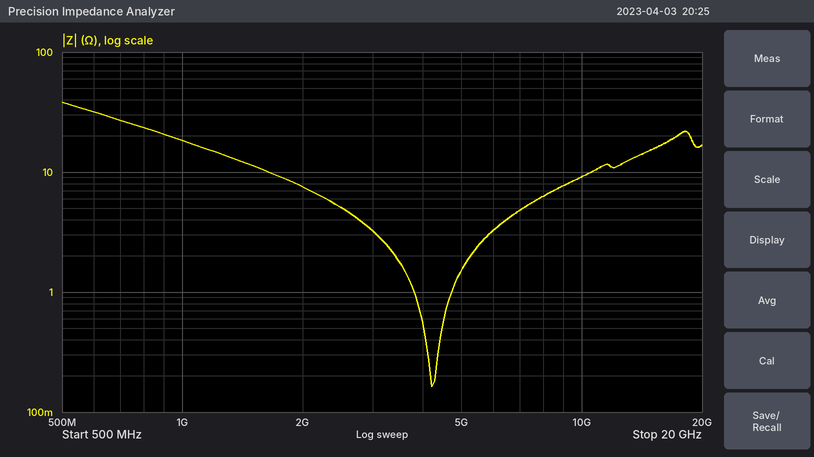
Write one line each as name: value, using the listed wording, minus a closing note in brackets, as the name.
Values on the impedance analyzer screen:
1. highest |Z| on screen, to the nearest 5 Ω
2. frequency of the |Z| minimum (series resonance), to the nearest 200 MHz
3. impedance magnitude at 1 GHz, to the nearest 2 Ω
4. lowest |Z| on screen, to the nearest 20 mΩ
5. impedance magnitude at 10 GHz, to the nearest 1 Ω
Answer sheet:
highest |Z| on screen, to the nearest 5 Ω: 40 Ω
frequency of the |Z| minimum (series resonance), to the nearest 200 MHz: 4.2 GHz
impedance magnitude at 1 GHz, to the nearest 2 Ω: 18 Ω
lowest |Z| on screen, to the nearest 20 mΩ: 160 mΩ
impedance magnitude at 10 GHz, to the nearest 1 Ω: 9 Ω
